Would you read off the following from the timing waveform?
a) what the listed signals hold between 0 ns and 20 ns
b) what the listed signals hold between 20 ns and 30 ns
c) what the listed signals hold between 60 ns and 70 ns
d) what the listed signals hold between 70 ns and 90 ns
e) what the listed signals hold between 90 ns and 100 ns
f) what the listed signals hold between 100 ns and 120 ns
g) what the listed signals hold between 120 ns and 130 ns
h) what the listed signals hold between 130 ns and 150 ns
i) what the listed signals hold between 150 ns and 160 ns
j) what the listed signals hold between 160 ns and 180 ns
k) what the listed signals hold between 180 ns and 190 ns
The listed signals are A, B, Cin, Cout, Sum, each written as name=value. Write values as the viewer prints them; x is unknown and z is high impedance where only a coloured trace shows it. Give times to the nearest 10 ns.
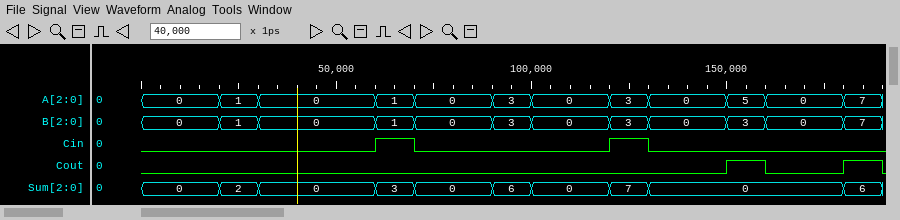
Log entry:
A=0, B=0, Cin=0, Cout=0, Sum=0
A=1, B=1, Cin=0, Cout=0, Sum=2
A=1, B=1, Cin=1, Cout=0, Sum=3
A=0, B=0, Cin=0, Cout=0, Sum=0
A=3, B=3, Cin=0, Cout=0, Sum=6
A=0, B=0, Cin=0, Cout=0, Sum=0
A=3, B=3, Cin=1, Cout=0, Sum=7
A=0, B=0, Cin=0, Cout=0, Sum=0
A=5, B=3, Cin=0, Cout=1, Sum=0
A=0, B=0, Cin=0, Cout=0, Sum=0
A=7, B=7, Cin=0, Cout=1, Sum=6
